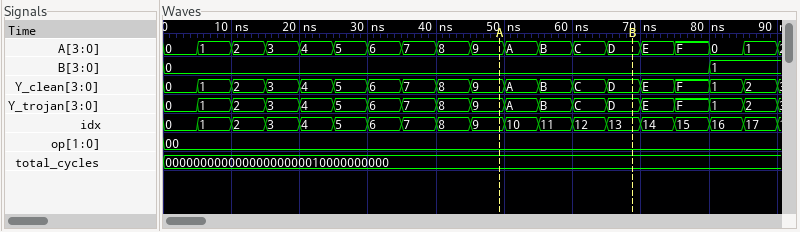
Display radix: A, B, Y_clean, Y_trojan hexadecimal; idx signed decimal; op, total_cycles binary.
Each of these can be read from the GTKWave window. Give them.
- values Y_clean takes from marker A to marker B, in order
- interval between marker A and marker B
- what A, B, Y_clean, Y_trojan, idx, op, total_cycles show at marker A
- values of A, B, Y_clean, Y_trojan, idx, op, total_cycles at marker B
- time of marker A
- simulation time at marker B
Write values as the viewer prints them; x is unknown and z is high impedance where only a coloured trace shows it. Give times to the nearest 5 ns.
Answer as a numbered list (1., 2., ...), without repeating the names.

1. 9, A, B, C, D
2. 20 ns
3. A=9, B=0, Y_clean=9, Y_trojan=9, idx=9, op=00, total_cycles=00000000000000000000010000000000
4. A=D, B=0, Y_clean=D, Y_trojan=D, idx=13, op=00, total_cycles=00000000000000000000010000000000
5. 50 ns
6. 70 ns
